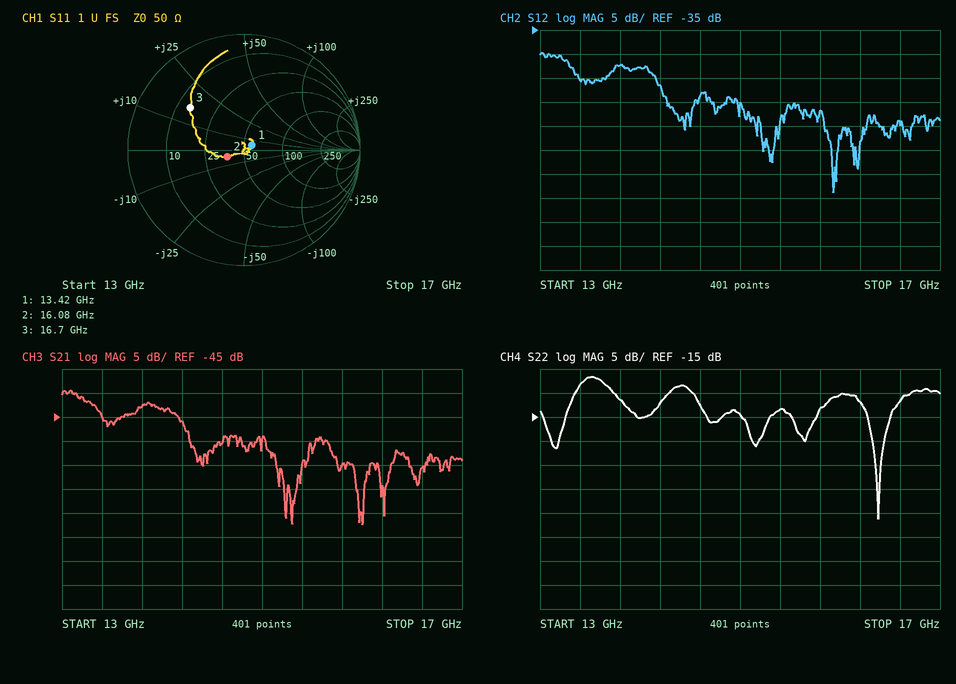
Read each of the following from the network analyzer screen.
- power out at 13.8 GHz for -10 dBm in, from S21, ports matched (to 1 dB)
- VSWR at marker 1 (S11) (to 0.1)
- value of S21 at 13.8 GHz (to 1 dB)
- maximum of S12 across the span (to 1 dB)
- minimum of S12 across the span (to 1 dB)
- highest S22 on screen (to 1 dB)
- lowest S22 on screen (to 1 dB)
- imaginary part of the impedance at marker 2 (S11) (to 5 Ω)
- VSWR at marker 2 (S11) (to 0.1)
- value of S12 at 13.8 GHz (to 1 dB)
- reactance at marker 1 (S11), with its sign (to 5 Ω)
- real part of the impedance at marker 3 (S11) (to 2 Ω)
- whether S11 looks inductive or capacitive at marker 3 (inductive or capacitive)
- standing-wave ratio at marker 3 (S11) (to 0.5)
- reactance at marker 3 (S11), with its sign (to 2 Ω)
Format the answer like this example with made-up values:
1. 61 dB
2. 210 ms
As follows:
1. -53 dBm
2. 1.2
3. -43 dB
4. -40 dB
5. -69 dB
6. -7 dB
7. -36 dB
8. -5 Ω
9. 1.4
10. -42 dB
11. +5 Ω
12. 14 Ω
13. inductive
14. 4.0
15. +16 Ω
